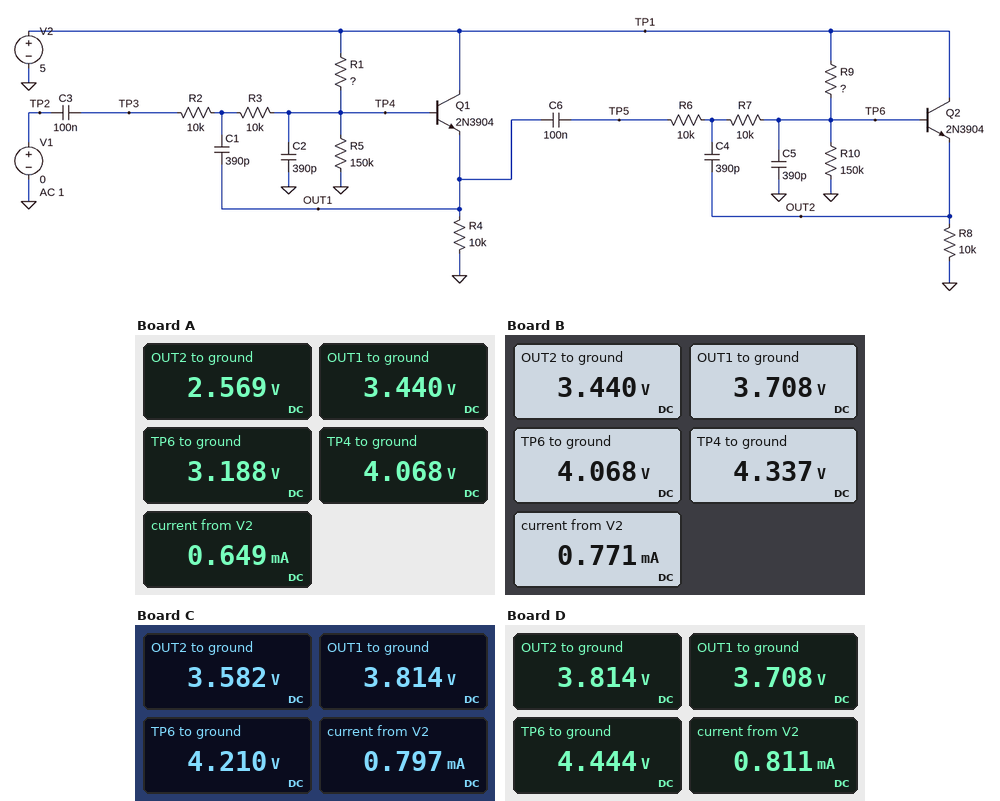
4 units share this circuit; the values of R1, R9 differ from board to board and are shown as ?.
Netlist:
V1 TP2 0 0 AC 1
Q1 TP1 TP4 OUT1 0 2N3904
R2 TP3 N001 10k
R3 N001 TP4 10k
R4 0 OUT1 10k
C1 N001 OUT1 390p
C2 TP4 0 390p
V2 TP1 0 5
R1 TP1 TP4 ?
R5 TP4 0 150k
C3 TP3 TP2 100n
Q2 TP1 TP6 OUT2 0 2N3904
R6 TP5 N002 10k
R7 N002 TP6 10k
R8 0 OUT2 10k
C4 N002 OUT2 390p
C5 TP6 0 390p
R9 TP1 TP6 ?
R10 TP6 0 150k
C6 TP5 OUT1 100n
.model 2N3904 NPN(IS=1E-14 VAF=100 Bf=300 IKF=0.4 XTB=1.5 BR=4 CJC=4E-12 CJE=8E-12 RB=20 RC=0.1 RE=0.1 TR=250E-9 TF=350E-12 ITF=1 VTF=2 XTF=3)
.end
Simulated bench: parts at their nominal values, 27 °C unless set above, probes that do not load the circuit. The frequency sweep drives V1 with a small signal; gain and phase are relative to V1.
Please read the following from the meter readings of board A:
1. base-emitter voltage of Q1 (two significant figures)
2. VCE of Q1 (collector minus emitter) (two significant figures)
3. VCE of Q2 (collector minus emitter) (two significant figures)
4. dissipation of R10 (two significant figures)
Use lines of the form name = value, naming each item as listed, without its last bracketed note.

base-emitter voltage of Q1 = 630 mV
VCE of Q1 (collector minus emitter) = 1.6 V
VCE of Q2 (collector minus emitter) = 2.4 V
dissipation of R10 = 68 µW
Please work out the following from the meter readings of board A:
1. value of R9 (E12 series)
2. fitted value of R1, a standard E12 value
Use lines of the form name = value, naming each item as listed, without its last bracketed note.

value of R9 = 82 kΩ
fitted value of R1, a standard E12 value = 33 kΩ
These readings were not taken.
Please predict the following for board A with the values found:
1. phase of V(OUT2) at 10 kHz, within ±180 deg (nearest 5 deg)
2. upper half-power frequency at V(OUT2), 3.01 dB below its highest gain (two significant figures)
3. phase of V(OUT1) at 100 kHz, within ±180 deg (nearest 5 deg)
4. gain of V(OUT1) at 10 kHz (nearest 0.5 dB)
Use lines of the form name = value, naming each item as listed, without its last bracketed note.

phase of V(OUT2) at 10 kHz, within ±180 deg = -40 deg
upper half-power frequency at V(OUT2), 3.01 dB below its highest gain = 25 kHz
phase of V(OUT1) at 100 kHz, within ±180 deg = -125 deg
gain of V(OUT1) at 10 kHz = -5.0 dB
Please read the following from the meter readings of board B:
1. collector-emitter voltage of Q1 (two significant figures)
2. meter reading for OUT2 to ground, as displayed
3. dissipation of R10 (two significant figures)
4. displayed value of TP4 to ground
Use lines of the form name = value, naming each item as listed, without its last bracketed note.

collector-emitter voltage of Q1 = 1.3 V
meter reading for OUT2 to ground, as displayed = 3.440 V
dissipation of R10 = 110 µW
displayed value of TP4 to ground = 4.337 V
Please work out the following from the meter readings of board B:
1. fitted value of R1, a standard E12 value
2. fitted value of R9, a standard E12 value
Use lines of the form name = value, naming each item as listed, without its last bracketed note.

fitted value of R1, a standard E12 value = 22 kΩ
fitted value of R9, a standard E12 value = 33 kΩ
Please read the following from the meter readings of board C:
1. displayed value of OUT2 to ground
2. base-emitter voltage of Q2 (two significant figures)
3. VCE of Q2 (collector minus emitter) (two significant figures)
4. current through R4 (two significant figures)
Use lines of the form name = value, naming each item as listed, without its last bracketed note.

displayed value of OUT2 to ground = 3.582 V
base-emitter voltage of Q2 = 630 mV
VCE of Q2 (collector minus emitter) = 1.4 V
current through R4 = 380 µA
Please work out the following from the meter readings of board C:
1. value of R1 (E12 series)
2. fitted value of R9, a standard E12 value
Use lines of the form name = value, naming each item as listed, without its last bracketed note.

value of R1 = 18 kΩ
fitted value of R9, a standard E12 value = 27 kΩ
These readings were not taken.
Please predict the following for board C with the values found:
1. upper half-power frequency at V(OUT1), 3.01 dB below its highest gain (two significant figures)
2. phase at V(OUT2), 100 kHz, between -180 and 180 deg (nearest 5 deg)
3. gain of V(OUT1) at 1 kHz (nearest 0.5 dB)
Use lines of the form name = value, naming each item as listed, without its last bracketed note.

upper half-power frequency at V(OUT1), 3.01 dB below its highest gain = 46 kHz
phase at V(OUT2), 100 kHz, between -180 and 180 deg = 120 deg
gain of V(OUT1) at 1 kHz = -7.0 dB
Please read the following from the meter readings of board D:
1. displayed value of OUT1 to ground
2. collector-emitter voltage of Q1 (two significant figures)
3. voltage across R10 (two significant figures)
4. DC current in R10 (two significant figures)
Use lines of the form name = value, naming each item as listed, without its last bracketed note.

displayed value of OUT1 to ground = 3.708 V
collector-emitter voltage of Q1 = 1.3 V
voltage across R10 = 4.4 V
DC current in R10 = 30 µA
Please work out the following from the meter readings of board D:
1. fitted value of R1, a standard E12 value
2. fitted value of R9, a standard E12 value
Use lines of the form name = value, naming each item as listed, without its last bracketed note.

fitted value of R1, a standard E12 value = 22 kΩ
fitted value of R9, a standard E12 value = 18 kΩ
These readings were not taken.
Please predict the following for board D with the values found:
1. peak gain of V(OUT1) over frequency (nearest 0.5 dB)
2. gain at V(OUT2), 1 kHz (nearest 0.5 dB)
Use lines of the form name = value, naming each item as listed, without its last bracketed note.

peak gain of V(OUT1) over frequency = -6.5 dB
gain at V(OUT2), 1 kHz = -13.5 dB
